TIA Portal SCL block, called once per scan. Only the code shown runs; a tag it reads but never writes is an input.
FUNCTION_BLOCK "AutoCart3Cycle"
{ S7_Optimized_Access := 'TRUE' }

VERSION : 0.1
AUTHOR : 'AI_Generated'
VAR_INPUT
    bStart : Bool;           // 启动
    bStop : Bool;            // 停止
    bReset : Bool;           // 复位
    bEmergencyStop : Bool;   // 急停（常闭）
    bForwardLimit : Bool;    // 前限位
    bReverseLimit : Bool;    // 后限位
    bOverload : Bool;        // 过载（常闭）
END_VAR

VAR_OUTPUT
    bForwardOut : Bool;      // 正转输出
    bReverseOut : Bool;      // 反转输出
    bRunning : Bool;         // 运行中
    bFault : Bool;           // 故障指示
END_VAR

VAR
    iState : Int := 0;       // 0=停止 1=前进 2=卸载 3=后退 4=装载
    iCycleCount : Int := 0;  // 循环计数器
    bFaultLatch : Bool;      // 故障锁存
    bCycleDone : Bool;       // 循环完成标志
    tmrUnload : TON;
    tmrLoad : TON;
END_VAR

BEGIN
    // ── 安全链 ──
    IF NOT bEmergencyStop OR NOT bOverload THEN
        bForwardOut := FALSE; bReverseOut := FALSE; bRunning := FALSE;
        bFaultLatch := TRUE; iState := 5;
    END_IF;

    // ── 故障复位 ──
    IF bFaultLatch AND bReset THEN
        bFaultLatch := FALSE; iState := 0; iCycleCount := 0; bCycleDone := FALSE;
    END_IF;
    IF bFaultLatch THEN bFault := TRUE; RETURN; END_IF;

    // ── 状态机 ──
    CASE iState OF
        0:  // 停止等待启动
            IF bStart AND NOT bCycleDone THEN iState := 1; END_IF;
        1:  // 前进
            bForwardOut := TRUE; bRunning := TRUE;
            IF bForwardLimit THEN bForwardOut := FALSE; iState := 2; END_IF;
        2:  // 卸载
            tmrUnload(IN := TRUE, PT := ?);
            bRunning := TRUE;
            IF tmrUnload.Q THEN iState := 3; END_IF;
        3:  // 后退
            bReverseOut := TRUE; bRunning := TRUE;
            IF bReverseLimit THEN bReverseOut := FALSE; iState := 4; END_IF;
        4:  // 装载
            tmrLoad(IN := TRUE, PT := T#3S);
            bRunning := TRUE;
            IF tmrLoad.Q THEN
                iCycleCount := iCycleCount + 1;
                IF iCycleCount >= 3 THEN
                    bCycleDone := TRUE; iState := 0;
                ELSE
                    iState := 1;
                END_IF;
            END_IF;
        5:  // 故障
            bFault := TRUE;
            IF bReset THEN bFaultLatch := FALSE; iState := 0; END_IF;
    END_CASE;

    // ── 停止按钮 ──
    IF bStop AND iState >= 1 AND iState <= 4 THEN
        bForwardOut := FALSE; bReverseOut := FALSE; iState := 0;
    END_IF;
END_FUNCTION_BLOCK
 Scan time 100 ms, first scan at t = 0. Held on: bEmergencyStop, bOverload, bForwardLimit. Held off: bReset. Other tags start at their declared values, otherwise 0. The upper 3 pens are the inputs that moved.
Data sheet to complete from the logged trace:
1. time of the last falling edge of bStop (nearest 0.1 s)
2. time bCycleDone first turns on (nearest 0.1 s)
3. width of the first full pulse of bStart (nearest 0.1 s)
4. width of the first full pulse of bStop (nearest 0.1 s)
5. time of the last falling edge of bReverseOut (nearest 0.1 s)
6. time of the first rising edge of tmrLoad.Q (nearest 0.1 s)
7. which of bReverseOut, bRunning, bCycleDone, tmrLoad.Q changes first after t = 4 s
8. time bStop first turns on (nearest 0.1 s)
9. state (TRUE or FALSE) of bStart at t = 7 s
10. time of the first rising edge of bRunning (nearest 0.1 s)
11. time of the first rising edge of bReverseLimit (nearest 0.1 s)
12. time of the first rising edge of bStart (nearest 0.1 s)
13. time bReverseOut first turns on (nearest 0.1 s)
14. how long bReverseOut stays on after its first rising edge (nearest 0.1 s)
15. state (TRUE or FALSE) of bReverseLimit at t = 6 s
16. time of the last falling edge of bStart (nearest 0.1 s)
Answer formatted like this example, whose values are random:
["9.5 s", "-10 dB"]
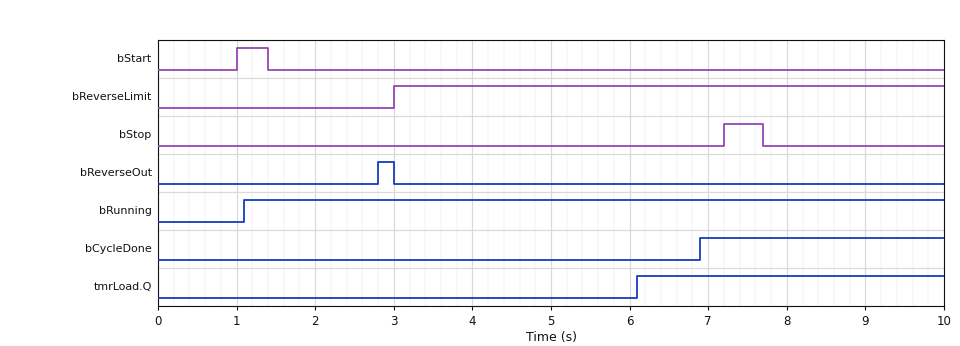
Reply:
["7.7 s", "6.9 s", "0.4 s", "0.5 s", "3.0 s", "6.1 s", "tmrLoad.Q", "7.2 s", "FALSE", "1.1 s", "3.0 s", "1.0 s", "2.8 s", "0.2 s", "TRUE", "1.4 s"]
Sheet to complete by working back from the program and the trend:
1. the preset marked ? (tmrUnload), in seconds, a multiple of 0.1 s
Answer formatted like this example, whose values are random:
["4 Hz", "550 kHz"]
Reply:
["1.5 s"]
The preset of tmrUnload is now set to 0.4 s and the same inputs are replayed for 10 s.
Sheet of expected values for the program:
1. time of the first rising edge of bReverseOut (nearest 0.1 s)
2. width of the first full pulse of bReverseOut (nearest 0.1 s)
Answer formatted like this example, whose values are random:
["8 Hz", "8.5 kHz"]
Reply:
["1.7 s", "1.3 s"]
